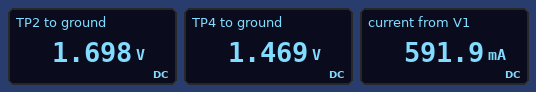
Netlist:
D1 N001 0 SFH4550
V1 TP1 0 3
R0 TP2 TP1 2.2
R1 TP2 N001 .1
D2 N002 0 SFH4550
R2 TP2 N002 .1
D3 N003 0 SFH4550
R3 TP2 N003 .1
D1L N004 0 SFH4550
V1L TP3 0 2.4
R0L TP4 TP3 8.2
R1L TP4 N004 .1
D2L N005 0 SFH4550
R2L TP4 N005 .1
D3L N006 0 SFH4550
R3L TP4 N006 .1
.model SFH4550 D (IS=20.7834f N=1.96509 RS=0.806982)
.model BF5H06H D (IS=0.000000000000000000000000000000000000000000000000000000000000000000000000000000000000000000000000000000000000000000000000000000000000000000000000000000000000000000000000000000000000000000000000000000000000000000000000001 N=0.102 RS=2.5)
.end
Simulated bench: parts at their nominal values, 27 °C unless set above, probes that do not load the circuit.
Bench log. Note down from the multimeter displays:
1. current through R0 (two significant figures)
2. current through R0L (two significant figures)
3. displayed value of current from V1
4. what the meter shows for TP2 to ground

590 mA
110 mA
591.9 mA
1.698 V
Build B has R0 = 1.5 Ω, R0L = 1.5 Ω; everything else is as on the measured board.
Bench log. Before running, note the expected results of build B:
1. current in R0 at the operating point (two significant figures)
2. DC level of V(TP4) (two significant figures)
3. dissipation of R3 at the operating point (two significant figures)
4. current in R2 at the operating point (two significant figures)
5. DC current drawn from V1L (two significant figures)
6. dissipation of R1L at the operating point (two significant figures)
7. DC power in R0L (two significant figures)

810 mA
1.7 V
7.3 mW
270 mA
490 mA
2.7 mW
370 mW
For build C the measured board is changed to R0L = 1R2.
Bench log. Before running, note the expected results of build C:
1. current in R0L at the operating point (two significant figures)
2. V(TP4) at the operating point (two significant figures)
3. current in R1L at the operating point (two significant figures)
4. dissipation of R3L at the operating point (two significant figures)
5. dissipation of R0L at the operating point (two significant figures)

590 mA
1.7 V
200 mA
3.8 mW
410 mW
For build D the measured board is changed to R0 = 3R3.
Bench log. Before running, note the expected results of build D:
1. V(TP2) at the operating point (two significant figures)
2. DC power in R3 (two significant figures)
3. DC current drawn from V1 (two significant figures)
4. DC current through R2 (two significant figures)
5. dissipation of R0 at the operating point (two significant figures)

1.6 V
1.9 mW
420 mA
140 mA
570 mW
